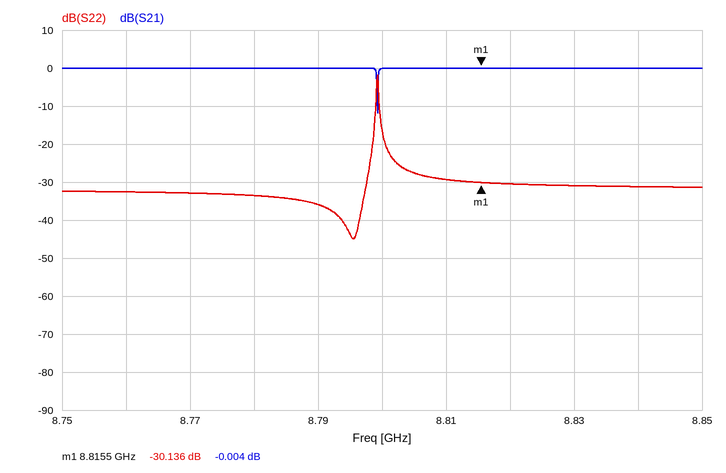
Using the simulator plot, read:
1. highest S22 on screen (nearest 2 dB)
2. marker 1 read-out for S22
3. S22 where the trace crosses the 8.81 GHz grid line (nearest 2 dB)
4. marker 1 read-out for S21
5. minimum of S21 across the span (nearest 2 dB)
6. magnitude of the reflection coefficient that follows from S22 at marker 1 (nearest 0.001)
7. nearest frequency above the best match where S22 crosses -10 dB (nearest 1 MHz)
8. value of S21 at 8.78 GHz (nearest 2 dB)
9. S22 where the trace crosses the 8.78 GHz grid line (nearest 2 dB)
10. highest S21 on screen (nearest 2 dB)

-2 dB
-30.136 dB
-30 dB
-0.004 dB
-12 dB
0.031
8.799 GHz
0 dB
-34 dB
0 dB
